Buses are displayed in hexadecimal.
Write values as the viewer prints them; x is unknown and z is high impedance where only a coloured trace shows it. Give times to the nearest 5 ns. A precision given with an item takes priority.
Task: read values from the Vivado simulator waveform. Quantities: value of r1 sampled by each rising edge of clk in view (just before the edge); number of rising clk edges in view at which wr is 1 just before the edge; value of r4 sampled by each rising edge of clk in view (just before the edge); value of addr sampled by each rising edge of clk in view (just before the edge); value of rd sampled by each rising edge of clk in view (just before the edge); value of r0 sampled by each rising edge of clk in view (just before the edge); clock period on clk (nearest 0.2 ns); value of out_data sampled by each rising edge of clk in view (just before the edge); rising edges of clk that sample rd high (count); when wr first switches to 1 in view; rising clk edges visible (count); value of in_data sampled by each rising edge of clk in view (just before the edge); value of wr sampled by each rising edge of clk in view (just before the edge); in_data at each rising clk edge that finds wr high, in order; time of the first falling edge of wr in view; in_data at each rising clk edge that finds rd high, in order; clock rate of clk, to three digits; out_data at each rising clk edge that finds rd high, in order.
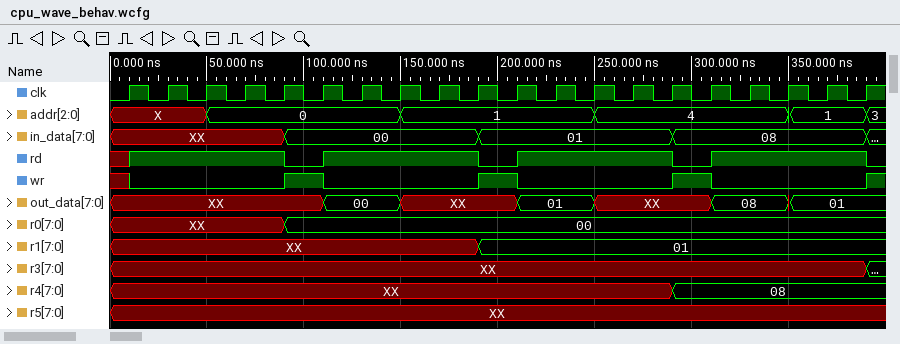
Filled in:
XX, XX, XX, XX, XX, XX, XX, XX, XX, XX, 01, 01, 01, 01, 01, 01, 01, 01, 01, 01
3
XX, XX, XX, XX, XX, XX, XX, XX, XX, XX, XX, XX, XX, XX, XX, 08, 08, 08, 08, 08
X, X, X, 0, 0, 0, 0, 0, 1, 1, 1, 1, 1, 4, 4, 4, 4, 4, 1, 1
x 1 1 1 1 0 1 1 1 1 0 1 1 1 1 0 1 1 1 1
XX, XX, XX, XX, XX, 00, 00, 00, 00, 00, 00, 00, 00, 00, 00, 00, 00, 00, 00, 00
20 ns
XX, XX, XX, XX, XX, XX, 00, 00, XX, XX, XX, 01, 01, XX, XX, XX, 08, 08, 01, 01
16
90 ns
20
XX, XX, XX, XX, XX, 00, 00, 00, 00, 00, 01, 01, 01, 01, 01, 08, 08, 08, 08, 08
x 0 0 0 0 1 0 0 0 0 1 0 0 0 0 1 0 0 0 0
00, 01, 08
110 ns
XX, XX, XX, XX, 00, 00, 00, 00, 01, 01, 01, 01, 08, 08, 08, 08
50.0 MHz
XX, XX, XX, XX, 00, 00, XX, XX, 01, 01, XX, XX, 08, 08, 01, 01
